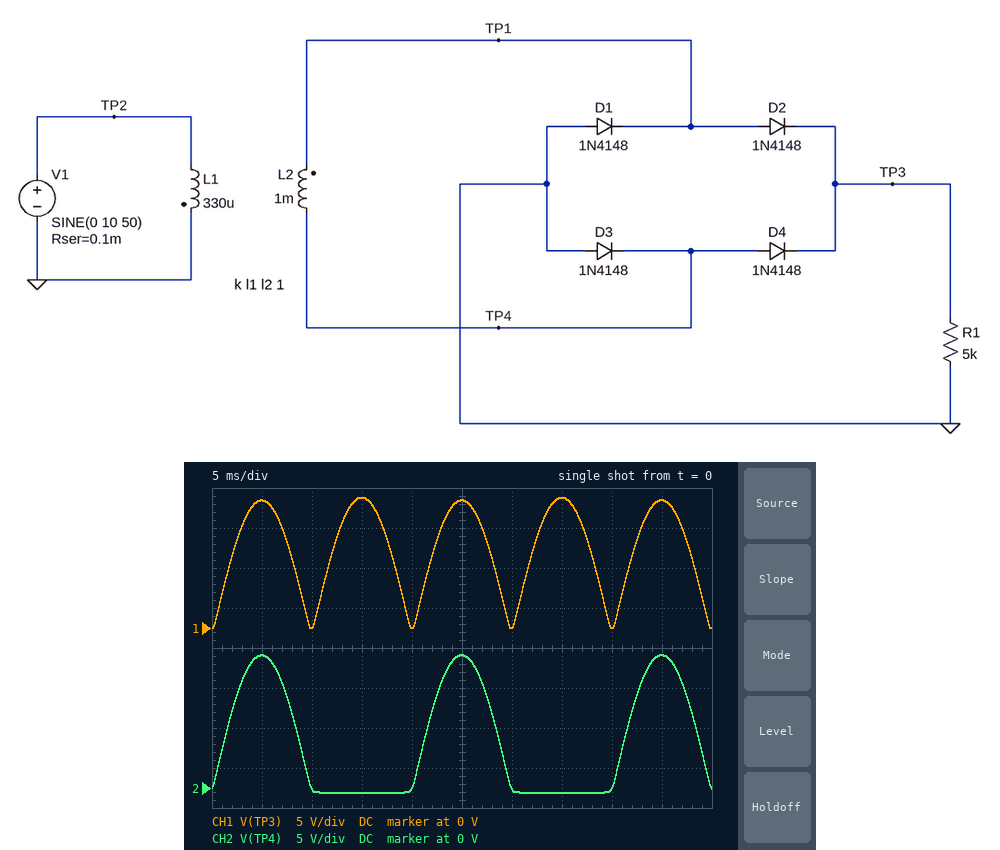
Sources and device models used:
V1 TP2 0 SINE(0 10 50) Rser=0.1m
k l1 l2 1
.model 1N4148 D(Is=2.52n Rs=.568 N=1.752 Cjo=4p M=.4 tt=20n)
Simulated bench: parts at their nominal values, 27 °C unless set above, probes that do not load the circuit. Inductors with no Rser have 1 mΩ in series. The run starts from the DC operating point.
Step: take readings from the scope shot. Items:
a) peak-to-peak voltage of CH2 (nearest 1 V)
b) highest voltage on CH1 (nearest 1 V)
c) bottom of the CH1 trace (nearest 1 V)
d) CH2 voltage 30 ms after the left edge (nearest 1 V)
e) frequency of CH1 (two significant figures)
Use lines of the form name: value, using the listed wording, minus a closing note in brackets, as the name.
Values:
peak-to-peak voltage of CH2: 17 V
highest voltage on CH1: 16 V
bottom of the CH1 trace: 0 V
CH2 voltage 30 ms after the left edge: 0 V
frequency of CH1: 100 Hz
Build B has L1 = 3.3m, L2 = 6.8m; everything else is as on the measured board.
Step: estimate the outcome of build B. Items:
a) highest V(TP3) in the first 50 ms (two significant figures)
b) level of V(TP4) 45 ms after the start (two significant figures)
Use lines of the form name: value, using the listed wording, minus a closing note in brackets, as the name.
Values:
highest V(TP3) in the first 50 ms: 13 V
level of V(TP4) 45 ms after the start: 14 V
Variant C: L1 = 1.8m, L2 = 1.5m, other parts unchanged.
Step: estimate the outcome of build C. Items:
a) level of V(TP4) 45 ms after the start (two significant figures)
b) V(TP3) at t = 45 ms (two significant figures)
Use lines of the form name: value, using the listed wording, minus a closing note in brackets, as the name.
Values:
level of V(TP4) 45 ms after the start: 8.5 V
V(TP3) at t = 45 ms: 7.9 V
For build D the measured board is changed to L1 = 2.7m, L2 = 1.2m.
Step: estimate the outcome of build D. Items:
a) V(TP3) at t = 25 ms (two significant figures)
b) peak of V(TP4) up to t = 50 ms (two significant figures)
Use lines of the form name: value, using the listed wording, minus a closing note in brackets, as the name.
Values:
V(TP3) at t = 25 ms: 5.5 V
peak of V(TP4) up to t = 50 ms: 6.1 V
